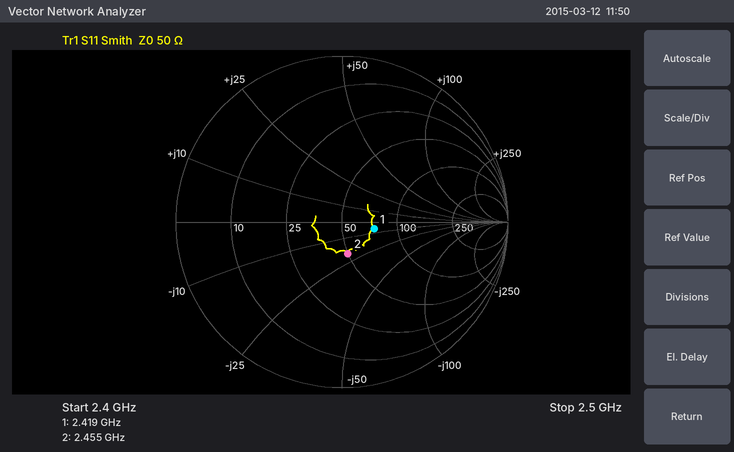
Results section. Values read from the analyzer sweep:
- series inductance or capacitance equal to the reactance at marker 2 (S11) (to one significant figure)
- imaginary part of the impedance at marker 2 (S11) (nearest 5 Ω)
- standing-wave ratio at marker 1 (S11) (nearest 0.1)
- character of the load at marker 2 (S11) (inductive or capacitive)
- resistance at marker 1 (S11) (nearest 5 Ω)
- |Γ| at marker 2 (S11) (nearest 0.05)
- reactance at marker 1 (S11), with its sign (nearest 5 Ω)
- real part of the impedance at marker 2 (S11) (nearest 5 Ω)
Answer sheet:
3 pF
-20 Ω
1.5
capacitive
75 Ω
0.20
-5 Ω
50 Ω
